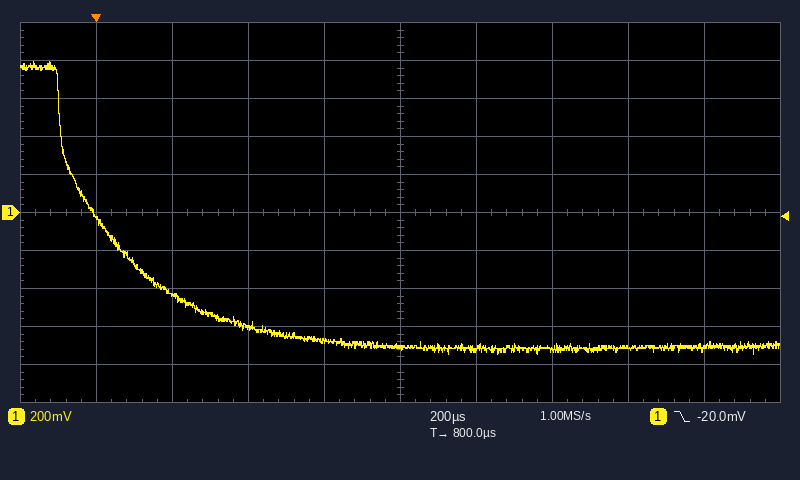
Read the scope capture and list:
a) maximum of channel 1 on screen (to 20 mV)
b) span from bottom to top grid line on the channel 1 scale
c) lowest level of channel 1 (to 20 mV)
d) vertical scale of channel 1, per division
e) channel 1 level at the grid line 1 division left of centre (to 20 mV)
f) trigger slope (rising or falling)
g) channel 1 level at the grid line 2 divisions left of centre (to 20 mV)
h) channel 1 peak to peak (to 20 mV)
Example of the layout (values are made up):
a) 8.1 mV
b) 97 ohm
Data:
a) 800 mV
b) 2 V
c) -740 mV
d) 200 mV
e) -680 mV
f) falling
g) -600 mV
h) 1.54 V
